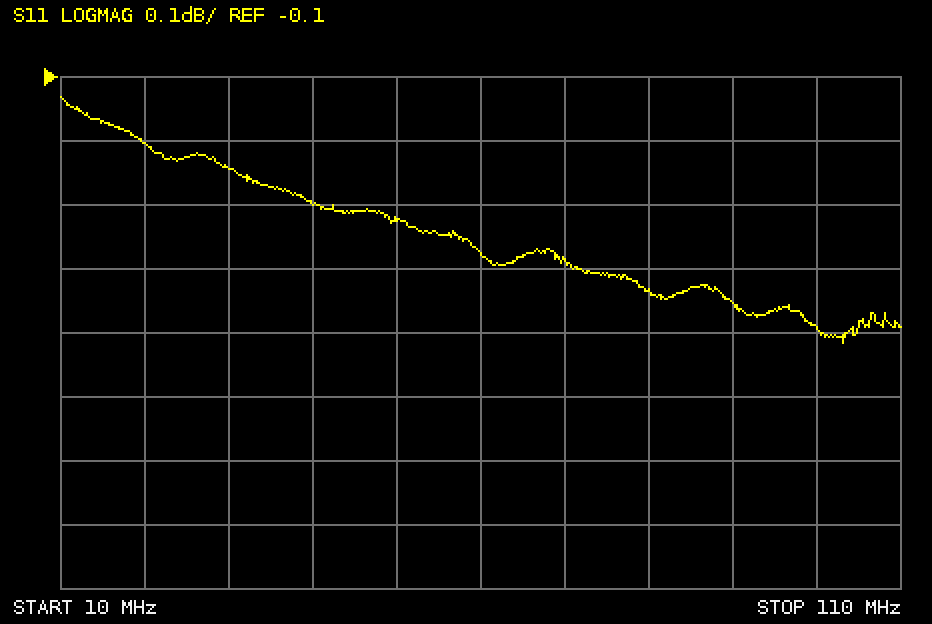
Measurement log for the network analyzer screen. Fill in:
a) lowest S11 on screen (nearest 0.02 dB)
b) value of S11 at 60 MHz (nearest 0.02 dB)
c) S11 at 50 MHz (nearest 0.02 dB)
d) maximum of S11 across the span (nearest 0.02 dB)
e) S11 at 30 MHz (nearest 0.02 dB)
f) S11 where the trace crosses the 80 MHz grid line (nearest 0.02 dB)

-0.52 dB
-0.38 dB
-0.32 dB
-0.14 dB
-0.24 dB
-0.44 dB
